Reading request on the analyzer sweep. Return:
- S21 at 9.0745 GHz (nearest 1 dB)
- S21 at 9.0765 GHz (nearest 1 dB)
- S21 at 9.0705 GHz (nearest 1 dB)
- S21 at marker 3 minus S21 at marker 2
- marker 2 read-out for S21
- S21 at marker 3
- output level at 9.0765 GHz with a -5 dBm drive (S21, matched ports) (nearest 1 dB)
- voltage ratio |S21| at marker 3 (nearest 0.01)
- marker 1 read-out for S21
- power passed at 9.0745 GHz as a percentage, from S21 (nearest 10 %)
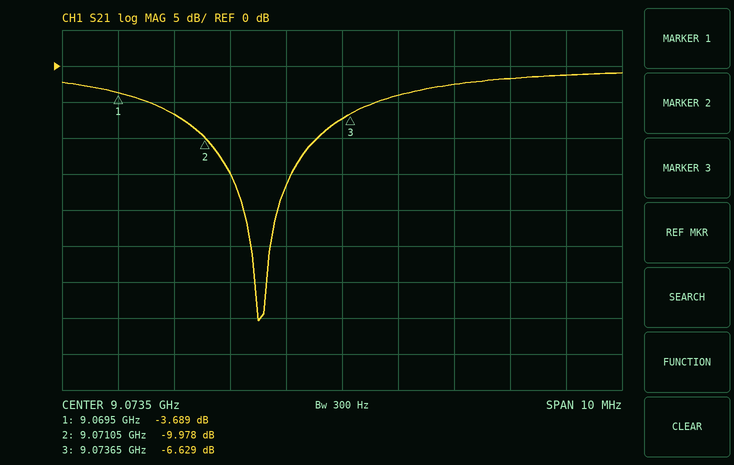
-4 dB
-2 dB
-7 dB
3.349 dB
-9.978 dB
-6.629 dB
-7 dBm
0.47
-3.689 dB
40 %
